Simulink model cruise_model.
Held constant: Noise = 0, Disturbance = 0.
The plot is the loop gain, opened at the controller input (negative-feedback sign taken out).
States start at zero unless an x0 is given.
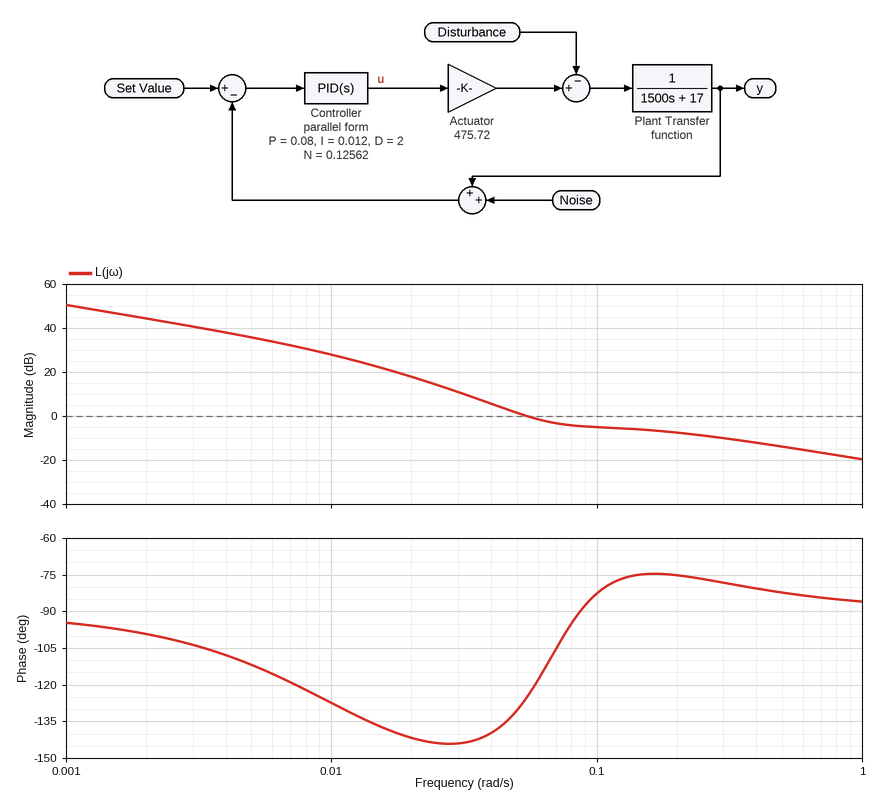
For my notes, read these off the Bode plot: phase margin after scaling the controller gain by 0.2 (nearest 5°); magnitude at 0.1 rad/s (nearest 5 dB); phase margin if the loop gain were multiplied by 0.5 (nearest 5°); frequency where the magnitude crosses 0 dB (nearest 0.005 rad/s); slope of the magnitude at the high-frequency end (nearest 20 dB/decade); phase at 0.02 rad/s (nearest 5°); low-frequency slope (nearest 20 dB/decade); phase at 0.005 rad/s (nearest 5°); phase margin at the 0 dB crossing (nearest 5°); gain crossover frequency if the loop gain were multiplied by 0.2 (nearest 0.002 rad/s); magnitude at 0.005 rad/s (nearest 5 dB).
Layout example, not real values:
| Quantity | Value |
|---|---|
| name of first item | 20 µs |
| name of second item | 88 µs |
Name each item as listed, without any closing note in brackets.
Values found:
| Quantity | Value |
|---|---|
| phase margin after scaling the controller gain by 0.2 | 35° |
| magnitude at 0.1 rad/s | -5 dB |
| phase margin if the loop gain were multiplied by 0.5 | 40° |
| frequency where the magnitude crosses 0 dB | 0.055 rad/s |
| slope of the magnitude at the high-frequency end | -20 dB/decade |
| phase at 0.02 rad/s | -140° |
| low-frequency slope | -20 dB/decade |
| phase at 0.005 rad/s | -110° |
| phase margin at the 0 dB crossing | 55° |
| gain crossover frequency if the loop gain were multiplied by 0.2 | 0.026 rad/s |
| magnitude at 0.005 rad/s | 35 dB |
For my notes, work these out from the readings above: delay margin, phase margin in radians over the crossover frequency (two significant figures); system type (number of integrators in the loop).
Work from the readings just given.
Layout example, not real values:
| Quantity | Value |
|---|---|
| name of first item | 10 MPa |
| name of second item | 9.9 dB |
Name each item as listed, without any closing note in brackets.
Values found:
| Quantity | Value |
|---|---|
| delay margin, phase margin in radians over the crossover frequency | 17 s |
| system type | 1 |
